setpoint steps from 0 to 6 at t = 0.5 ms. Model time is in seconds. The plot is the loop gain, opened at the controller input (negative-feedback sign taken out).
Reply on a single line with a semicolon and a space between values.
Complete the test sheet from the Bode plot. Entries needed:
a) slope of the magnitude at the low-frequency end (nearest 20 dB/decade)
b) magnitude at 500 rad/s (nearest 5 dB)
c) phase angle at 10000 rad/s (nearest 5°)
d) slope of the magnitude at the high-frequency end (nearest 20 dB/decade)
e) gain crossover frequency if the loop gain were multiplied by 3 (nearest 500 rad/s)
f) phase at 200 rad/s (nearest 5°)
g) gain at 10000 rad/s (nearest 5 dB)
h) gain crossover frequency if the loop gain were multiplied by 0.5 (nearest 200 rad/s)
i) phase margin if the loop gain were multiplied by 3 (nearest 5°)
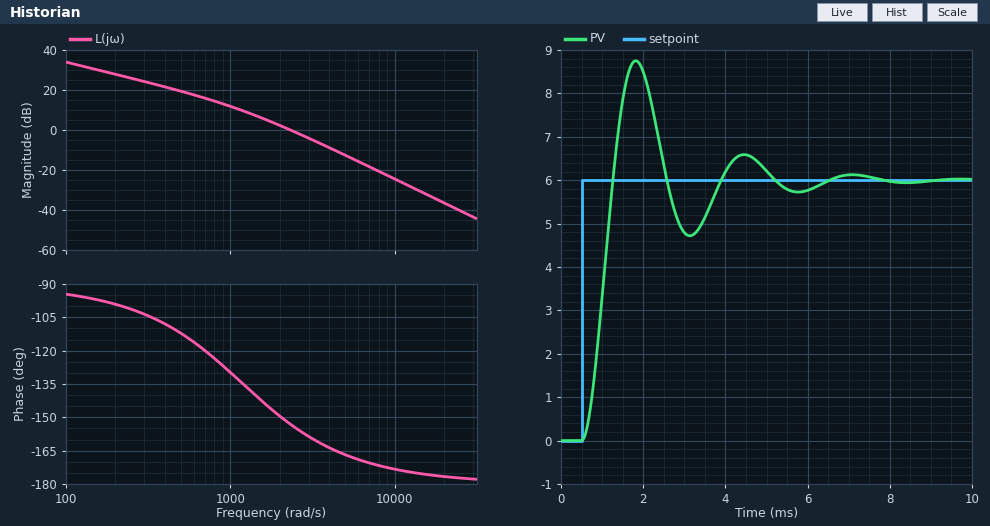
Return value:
-20 dB/decade; 20 dB; -175°; -40 dB/decade; 4000 rad/s; -100°; -25 dB; 1600 rad/s; 15°
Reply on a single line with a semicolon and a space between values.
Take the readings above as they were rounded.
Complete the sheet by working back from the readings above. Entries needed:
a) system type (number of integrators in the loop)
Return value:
1
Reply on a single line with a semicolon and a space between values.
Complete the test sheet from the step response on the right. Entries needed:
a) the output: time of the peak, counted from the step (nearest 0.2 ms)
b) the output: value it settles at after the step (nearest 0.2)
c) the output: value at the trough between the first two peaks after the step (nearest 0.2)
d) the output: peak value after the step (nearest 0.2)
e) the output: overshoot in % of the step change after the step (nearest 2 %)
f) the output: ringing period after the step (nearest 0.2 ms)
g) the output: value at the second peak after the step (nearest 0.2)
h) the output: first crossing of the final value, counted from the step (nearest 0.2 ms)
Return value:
1.4 ms; 6.0; 4.8; 8.8; 46 %; 2.6 ms; 6.6; 0.8 ms
